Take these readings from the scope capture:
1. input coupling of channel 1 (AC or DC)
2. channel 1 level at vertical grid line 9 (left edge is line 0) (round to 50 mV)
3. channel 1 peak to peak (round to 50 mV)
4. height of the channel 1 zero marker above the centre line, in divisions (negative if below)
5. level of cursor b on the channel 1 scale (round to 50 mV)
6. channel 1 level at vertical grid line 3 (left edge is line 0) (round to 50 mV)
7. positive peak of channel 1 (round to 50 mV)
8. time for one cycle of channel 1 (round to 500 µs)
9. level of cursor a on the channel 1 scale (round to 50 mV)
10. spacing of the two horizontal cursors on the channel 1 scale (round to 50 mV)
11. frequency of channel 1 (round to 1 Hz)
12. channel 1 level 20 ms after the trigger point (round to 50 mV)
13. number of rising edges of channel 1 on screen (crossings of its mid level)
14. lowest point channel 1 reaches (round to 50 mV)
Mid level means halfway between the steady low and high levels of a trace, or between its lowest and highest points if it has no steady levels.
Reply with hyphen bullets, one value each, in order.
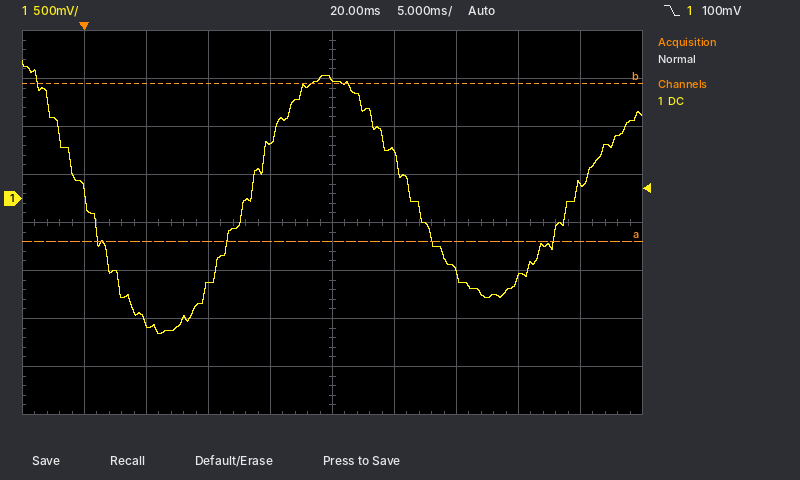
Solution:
- DC
- 150 mV
- 2.85 V
- +0.5 div
- 1.20 V
- -900 mV
- 1.45 V
- 26.0 ms
- -450 mV
- 1.65 V
- 38 Hz
- 1.25 V
- 2
- -1.40 V
